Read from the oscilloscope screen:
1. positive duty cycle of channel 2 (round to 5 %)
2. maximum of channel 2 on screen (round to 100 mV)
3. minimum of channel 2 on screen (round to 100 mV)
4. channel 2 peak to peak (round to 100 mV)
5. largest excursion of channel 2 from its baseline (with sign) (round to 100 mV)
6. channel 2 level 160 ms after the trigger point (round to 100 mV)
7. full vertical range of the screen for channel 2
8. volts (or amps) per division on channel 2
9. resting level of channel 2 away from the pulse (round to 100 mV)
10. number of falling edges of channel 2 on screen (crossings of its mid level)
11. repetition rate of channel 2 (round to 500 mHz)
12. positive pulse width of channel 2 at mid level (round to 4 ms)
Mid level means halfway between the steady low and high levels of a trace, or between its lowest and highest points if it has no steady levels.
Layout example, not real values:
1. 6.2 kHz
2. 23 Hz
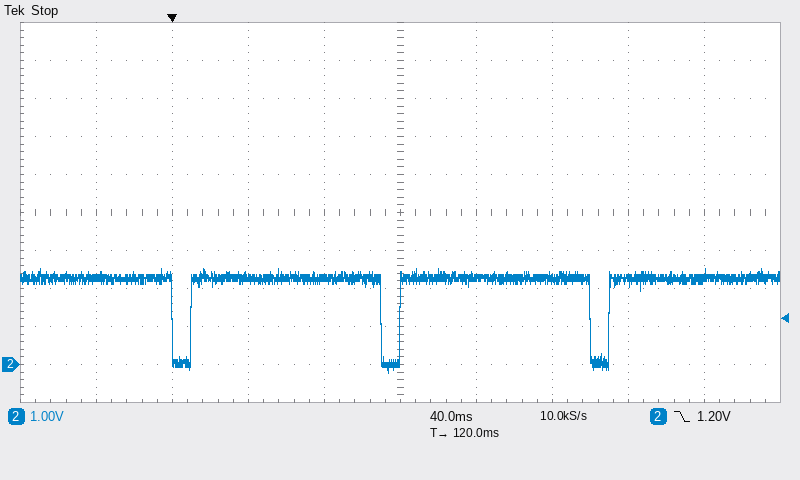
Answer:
1. 90 %
2. 2.5 V
3. -200 mV
4. 2.7 V
5. -2.5 V
6. 2.3 V
7. 10 V
8. 1 V
9. 2.3 V
10. 3
11. 9.0 Hz
12. 100 ms
